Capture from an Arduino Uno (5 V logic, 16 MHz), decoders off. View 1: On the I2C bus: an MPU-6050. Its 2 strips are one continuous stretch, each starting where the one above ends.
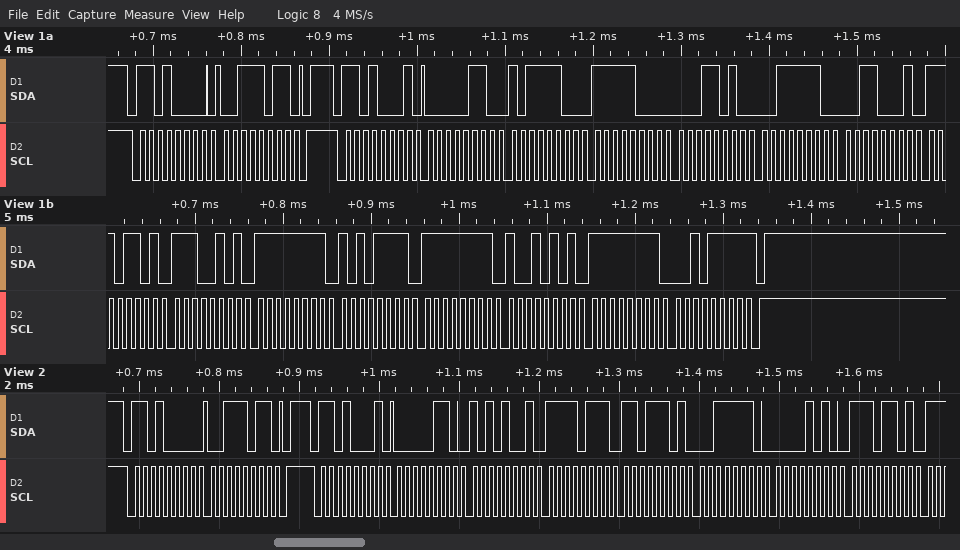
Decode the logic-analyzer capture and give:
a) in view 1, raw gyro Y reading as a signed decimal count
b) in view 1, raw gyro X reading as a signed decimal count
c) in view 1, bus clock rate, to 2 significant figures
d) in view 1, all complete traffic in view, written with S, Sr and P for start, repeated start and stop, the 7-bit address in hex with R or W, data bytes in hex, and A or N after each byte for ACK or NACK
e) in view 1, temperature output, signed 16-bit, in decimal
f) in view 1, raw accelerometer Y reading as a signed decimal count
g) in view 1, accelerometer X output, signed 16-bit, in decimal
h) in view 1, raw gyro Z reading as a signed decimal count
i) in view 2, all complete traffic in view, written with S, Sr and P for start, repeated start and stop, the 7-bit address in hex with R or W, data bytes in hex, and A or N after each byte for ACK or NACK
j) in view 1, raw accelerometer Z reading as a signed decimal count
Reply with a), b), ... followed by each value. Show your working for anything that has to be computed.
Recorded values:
a) 0xFF95 = -107
b) 0xFFAF = -81
c) 100 kHz
d) S 68W A 3B A P S 68R A 06 A BC A F8 A 1A A 3E A 31 A ED A E5 A FF A AF A FF A 95 A FF A 2F N P
e) 0xEDE5 = -4635
f) 0xF81A = -2022
g) 0x06BC = 1724
h) 0xFF2F = -209
i) S 68W A 3B A P S 68R A 06 A A9 A F7 A DD A 3E A 0A A ED A
j) 0x3E31 = 15921
